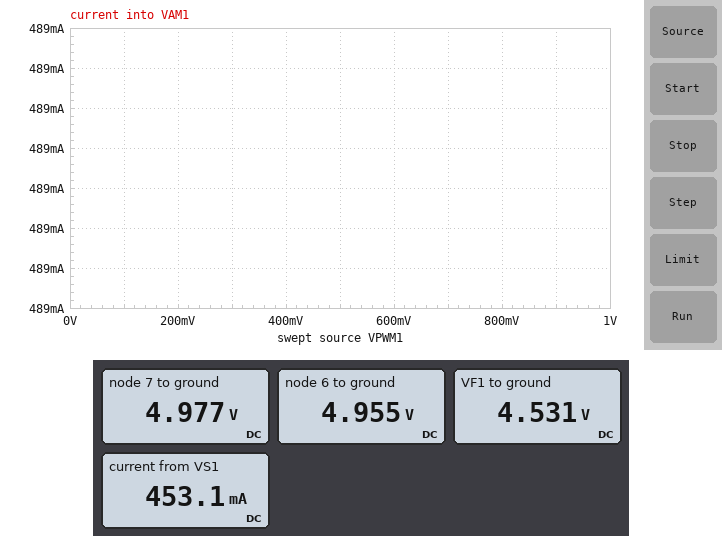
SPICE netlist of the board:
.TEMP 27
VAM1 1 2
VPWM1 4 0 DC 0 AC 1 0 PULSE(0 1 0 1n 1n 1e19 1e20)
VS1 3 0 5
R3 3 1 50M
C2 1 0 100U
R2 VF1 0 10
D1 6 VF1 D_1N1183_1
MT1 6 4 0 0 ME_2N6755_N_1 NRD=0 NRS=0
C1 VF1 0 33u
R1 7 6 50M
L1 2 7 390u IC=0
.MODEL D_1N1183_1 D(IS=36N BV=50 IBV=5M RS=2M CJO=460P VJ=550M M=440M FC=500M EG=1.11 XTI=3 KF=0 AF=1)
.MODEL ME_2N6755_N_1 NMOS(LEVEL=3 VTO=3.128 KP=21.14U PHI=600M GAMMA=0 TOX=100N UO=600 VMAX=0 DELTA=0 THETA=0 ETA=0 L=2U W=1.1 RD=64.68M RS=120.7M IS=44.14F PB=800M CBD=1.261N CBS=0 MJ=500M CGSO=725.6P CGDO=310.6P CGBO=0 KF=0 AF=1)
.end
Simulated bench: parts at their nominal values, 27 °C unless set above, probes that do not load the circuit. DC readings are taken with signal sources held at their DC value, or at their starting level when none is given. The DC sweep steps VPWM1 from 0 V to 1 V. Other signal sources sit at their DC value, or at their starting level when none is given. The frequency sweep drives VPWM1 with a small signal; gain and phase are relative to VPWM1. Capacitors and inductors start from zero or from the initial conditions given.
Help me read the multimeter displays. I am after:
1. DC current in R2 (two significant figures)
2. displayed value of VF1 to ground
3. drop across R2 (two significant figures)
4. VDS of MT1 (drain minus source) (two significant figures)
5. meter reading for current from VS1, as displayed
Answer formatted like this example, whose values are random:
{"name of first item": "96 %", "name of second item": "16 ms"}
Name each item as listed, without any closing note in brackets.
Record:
{"DC current in R2": "450 mA", "displayed value of VF1 to ground": "4.531 V", "drop across R2": "4.5 V", "VDS of MT1 (drain minus source)": "5.0 V", "meter reading for current from VS1, as displayed": "453.1 mA"}
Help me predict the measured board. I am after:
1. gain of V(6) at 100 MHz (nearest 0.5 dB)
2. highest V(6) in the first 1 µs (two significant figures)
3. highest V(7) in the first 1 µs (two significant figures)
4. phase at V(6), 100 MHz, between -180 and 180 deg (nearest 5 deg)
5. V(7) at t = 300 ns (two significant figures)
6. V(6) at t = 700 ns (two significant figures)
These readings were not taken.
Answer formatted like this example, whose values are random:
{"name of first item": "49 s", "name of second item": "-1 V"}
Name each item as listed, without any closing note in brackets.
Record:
{"gain of V(6) at 100 MHz": "-38.0 dB", "highest V(6) in the first 1 µs": "240 mV", "highest V(7) in the first 1 µs": "240 mV", "phase at V(6), 100 MHz, between -180 and 180 deg": "85 deg", "V(7) at t = 300 ns": "160 mV", "V(6) at t = 700 ns": "180 mV"}
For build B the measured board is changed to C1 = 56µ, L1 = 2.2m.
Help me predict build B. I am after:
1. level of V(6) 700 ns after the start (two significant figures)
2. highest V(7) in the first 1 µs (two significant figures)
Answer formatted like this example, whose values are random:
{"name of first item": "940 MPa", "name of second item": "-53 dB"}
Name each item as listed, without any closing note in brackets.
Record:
{"level of V(6) 700 ns after the start": "160 mV", "highest V(7) in the first 1 µs": "170 mV"}
